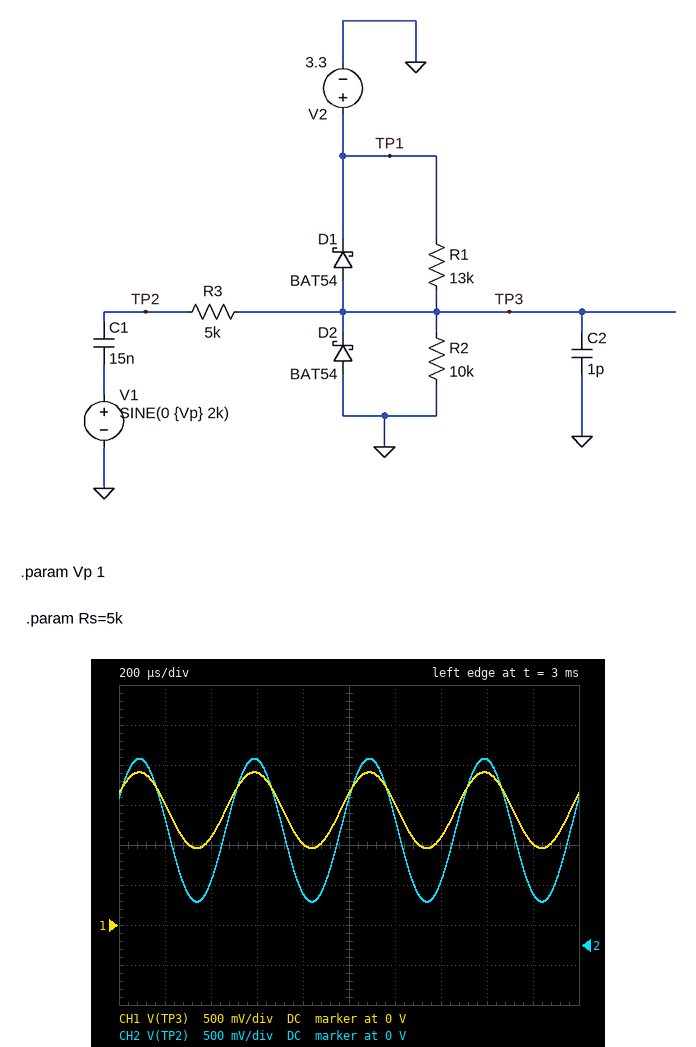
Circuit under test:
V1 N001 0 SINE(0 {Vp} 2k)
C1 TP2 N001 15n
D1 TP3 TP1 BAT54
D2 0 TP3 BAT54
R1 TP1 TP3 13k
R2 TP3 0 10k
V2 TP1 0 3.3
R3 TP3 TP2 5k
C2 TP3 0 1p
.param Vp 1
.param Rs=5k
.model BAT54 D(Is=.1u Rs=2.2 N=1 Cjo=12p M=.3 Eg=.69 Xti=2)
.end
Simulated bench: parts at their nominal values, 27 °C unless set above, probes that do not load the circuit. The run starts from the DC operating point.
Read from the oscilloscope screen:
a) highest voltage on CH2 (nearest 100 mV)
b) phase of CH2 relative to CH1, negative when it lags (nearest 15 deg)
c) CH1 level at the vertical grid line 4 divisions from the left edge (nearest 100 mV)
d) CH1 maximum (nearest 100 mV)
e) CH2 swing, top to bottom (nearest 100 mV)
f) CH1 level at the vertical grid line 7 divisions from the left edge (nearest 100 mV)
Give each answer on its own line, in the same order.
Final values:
2.3 V
0 deg
1.0 V
1.9 V
1.8 V
1.1 V
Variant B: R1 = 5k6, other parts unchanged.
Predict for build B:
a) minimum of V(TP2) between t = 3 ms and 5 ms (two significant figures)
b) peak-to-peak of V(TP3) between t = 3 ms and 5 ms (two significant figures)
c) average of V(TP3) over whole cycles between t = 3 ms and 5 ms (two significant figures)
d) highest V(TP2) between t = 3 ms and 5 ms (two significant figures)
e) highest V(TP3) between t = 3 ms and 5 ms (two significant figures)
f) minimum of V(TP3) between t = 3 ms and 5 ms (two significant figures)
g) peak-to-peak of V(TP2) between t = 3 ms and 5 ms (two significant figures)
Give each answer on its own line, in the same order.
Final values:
1.3 V
710 mV
2.1 V
3.0 V
2.5 V
1.8 V
1.7 V
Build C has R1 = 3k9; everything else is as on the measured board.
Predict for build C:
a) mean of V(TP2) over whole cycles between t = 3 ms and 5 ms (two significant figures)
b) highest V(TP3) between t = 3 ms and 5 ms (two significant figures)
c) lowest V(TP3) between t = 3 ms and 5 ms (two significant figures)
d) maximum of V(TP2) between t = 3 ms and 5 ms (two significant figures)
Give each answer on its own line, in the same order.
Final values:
2.4 V
2.7 V
2.1 V
3.2 V
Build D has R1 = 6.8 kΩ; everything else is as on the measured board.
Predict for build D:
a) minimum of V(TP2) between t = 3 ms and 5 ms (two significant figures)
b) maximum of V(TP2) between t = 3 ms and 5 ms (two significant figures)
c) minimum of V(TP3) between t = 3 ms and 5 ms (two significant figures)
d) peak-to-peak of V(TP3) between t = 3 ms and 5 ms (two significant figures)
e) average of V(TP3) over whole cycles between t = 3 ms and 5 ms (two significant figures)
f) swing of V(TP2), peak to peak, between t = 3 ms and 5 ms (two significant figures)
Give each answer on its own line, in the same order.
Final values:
1.1 V
2.8 V
1.6 V
770 mV
2.0 V
1.7 V
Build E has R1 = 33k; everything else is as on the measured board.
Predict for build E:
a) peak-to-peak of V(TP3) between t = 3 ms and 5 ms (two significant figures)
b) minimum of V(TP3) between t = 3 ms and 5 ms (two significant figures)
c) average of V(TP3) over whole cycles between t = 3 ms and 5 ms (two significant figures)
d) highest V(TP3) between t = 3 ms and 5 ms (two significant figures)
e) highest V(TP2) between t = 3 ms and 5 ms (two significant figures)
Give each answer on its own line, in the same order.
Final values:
1.1 V
210 mV
770 mV
1.3 V
1.7 V
